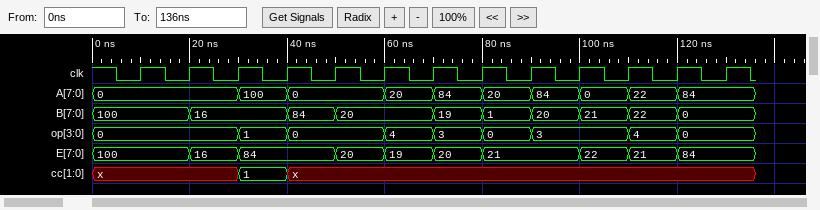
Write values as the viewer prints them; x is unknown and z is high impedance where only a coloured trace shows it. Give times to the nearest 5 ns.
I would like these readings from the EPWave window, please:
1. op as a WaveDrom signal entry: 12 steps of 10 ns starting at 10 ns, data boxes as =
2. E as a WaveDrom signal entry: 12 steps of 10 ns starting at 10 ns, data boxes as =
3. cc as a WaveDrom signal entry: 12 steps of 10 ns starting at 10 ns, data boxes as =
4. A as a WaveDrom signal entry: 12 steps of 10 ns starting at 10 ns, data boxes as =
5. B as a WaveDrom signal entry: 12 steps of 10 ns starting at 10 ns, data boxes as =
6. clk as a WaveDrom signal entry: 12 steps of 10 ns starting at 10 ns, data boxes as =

{name: 'op', wave: '=.==.====.==', data: '0 1 0 4 3 0 3 4 0'}
{name: 'E', wave: '===.====.===', data: '100 16 84 20 19 20 21 22 21 84'}
{name: 'cc', wave: 'x.=x........', data: '1'}
{name: 'A', wave: '=.==.=======', data: '0 100 0 20 84 20 84 0 22 84'}
{name: 'B', wave: '==.==.======', data: '100 16 84 20 19 1 20 21 22 0'}
{name: 'clk', wave: 'p...........'}
